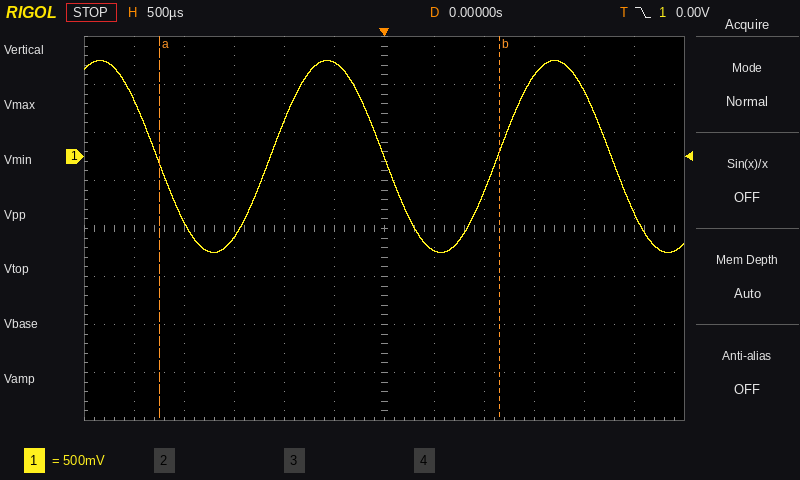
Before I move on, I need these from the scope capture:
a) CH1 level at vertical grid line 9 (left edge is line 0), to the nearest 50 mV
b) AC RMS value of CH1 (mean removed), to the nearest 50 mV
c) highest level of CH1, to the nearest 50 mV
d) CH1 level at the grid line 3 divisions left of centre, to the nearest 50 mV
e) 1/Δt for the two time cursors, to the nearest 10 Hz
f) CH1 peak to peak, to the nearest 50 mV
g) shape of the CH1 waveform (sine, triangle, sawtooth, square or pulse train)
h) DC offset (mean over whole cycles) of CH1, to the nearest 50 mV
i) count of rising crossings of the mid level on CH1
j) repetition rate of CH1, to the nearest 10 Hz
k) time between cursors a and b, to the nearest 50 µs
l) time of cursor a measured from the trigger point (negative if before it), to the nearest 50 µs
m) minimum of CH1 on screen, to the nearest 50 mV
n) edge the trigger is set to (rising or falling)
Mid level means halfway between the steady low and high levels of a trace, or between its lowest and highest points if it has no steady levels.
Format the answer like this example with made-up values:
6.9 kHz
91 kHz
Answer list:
850 mV
700 mV
1.00 V
-850 mV
290 Hz
2.00 V
sine
0 mV
2
440 Hz
3.40 ms
-2.25 ms
-1.00 V
falling
